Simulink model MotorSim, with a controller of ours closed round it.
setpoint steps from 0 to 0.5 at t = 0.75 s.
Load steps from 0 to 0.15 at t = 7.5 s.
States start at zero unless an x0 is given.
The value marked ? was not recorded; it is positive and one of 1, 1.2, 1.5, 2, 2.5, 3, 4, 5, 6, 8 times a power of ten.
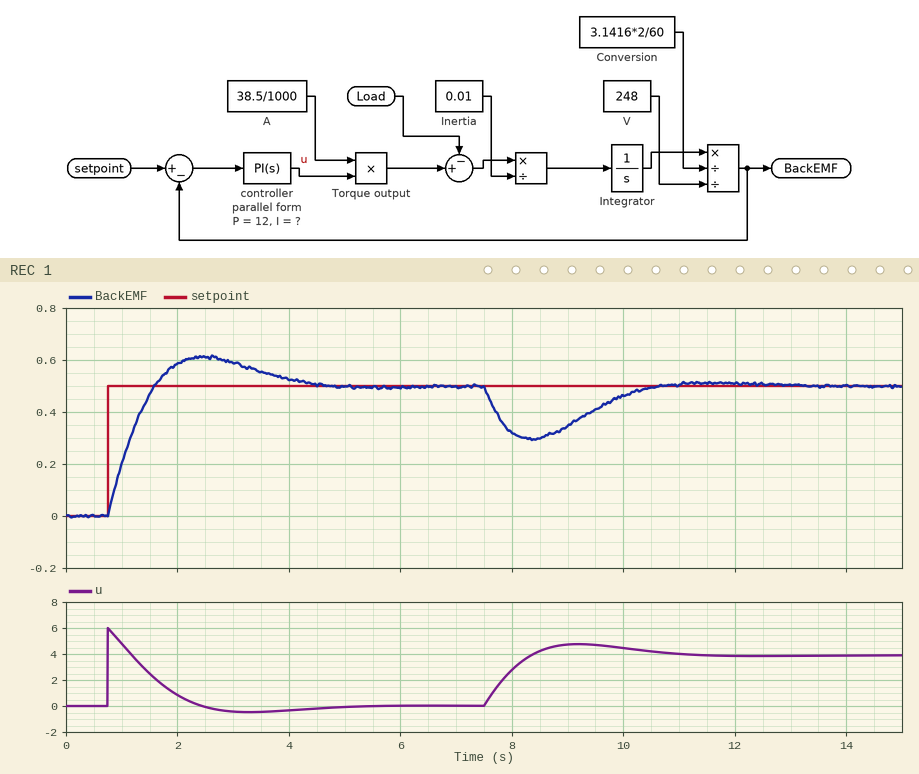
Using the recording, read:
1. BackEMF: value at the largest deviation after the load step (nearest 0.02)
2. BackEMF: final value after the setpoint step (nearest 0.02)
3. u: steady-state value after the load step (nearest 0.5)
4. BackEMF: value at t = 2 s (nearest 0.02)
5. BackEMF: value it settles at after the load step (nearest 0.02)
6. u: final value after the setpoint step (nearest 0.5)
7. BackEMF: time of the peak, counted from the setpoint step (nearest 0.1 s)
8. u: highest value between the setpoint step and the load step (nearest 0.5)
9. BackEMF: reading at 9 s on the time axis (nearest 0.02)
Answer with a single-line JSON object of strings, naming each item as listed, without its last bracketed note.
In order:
{"BackEMF: value at the largest deviation after the load step": "0.30", "BackEMF: final value after the setpoint step": "0.50", "u: steady-state value after the load step": "4.0", "BackEMF: value at t = 2 s": "0.58", "BackEMF: value it settles at after the load step": "0.50", "u: final value after the setpoint step": "0.0", "BackEMF: time of the peak, counted from the setpoint step": "1.7 s", "u: highest value between the setpoint step and the load step": "6.0", "BackEMF: reading at 9 s on the time axis": "0.34"}
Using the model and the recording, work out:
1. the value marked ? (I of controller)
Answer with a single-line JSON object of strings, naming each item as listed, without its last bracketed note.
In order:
{"the value marked ?": "12"}
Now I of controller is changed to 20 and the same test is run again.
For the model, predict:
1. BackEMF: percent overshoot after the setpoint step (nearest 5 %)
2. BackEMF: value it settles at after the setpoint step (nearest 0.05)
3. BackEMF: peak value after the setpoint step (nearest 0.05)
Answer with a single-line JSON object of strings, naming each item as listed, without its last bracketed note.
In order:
{"BackEMF: percent overshoot after the setpoint step": "30 %", "BackEMF: value it settles at after the setpoint step": "0.50", "BackEMF: peak value after the setpoint step": "0.65"}
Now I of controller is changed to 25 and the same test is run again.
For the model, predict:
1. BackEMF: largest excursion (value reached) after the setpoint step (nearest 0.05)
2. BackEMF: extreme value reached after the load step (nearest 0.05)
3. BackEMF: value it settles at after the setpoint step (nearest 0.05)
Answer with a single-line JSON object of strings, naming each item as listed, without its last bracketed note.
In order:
{"BackEMF: largest excursion (value reached) after the setpoint step": "0.65", "BackEMF: extreme value reached after the load step": "0.35", "BackEMF: value it settles at after the setpoint step": "0.50"}
